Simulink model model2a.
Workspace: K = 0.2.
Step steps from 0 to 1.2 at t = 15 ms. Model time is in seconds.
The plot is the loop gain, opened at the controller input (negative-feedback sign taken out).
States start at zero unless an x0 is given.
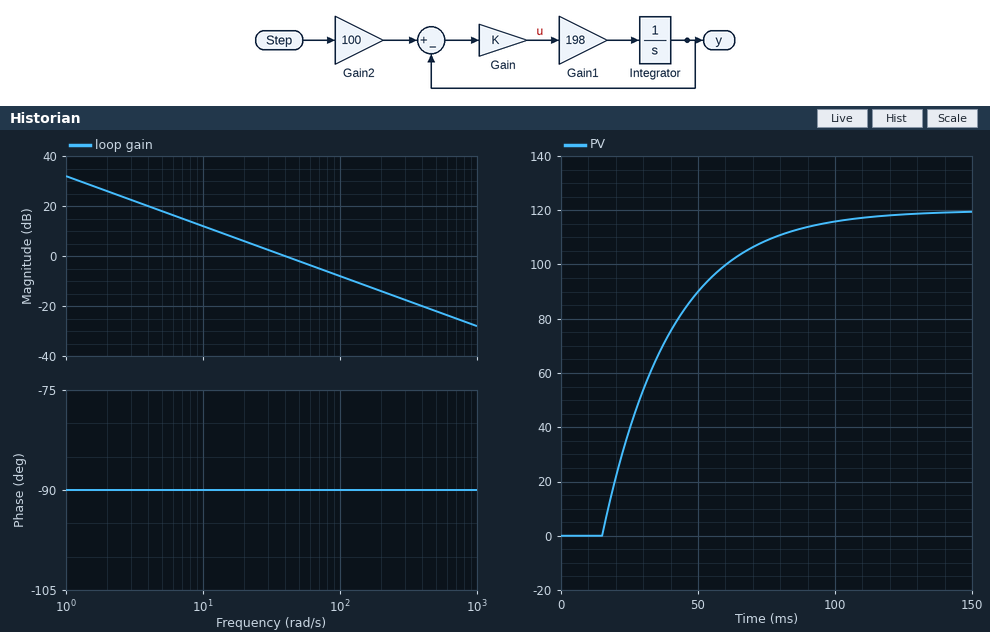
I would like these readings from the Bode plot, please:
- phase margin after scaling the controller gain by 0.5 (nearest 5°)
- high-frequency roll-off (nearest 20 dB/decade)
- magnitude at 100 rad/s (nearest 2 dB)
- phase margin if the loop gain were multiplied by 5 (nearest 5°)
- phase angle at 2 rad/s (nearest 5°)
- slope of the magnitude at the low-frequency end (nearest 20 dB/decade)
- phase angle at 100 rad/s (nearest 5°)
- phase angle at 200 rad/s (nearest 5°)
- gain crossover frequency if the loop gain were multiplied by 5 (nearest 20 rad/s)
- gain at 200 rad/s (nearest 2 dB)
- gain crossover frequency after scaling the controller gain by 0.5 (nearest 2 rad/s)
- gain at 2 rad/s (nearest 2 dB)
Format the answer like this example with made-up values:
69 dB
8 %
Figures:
90°
-20 dB/decade
-8 dB
90°
-90°
-20 dB/decade
-90°
-90°
200 rad/s
-14 dB
20 rad/s
26 dB
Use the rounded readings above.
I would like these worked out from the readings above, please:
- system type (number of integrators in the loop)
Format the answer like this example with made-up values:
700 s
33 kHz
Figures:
1
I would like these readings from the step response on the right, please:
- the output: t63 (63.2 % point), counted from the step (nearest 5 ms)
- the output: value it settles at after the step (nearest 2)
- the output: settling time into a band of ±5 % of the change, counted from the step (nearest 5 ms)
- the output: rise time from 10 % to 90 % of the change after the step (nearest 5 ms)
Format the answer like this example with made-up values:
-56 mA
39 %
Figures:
25 ms
120
75 ms
55 ms
